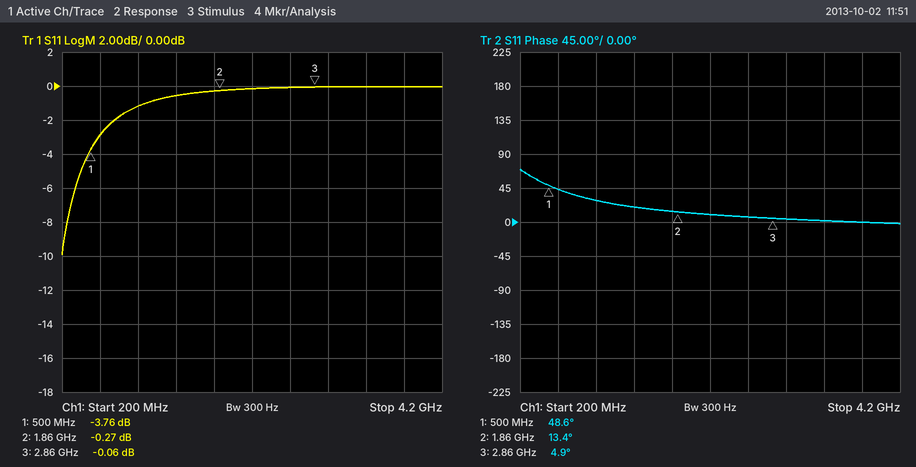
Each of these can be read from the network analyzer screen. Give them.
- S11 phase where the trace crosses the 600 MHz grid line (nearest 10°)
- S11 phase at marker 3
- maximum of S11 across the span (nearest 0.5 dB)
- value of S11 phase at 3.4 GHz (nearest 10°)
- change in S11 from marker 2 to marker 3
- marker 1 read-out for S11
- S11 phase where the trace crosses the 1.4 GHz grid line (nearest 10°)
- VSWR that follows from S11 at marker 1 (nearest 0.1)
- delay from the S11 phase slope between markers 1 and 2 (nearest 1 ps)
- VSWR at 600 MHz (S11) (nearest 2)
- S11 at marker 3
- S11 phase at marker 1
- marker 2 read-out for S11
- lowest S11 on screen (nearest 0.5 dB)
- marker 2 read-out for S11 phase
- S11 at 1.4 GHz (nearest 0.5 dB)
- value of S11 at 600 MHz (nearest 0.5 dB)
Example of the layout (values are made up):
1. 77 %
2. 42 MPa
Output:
1. 40°
2. 4.9°
3. 0.0 dB
4. 0°
5. 0.21 dB
6. -3.76 dB
7. 20°
8. 4.7
9. 72 ps
10. 6
11. -0.06 dB
12. 48.6°
13. -0.27 dB
14. -10.0 dB
15. 13.4°
16. -0.5 dB
17. -3.0 dB
